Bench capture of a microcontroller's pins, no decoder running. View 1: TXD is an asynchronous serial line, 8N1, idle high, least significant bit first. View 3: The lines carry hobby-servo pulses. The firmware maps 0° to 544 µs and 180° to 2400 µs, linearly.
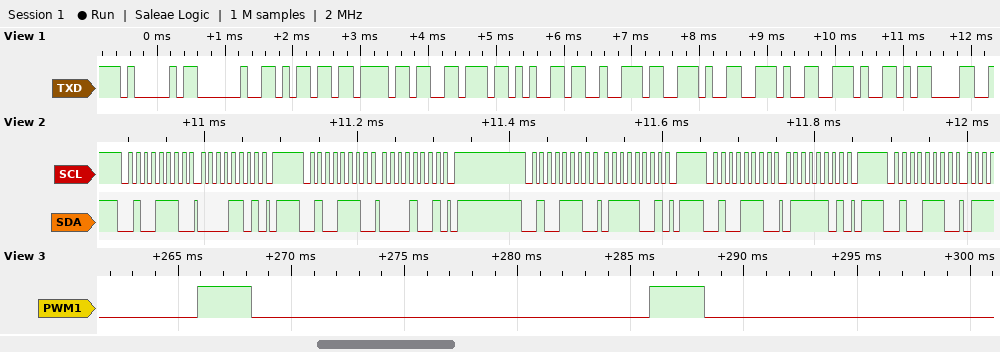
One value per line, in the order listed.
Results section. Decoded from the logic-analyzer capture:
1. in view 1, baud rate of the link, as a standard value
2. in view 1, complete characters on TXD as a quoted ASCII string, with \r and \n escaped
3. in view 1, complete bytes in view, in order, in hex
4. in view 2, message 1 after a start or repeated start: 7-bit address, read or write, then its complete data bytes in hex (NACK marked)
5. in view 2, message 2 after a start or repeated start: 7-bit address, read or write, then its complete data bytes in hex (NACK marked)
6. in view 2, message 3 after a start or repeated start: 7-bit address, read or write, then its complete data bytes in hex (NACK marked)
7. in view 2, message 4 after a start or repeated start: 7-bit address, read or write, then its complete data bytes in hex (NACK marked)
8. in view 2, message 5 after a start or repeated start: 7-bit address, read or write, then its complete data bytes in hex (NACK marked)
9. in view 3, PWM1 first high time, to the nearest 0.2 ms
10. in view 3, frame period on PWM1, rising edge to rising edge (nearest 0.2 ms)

9600 baud
"A mover...\r"
41 20 6D 6F 76 65 72 2E 2E 2E 0D
0x27 write: 0D
0x27 write: 09
0x27 write: 79
0x27 write: 7D
0x27 write
2.4 ms
20.0 ms
